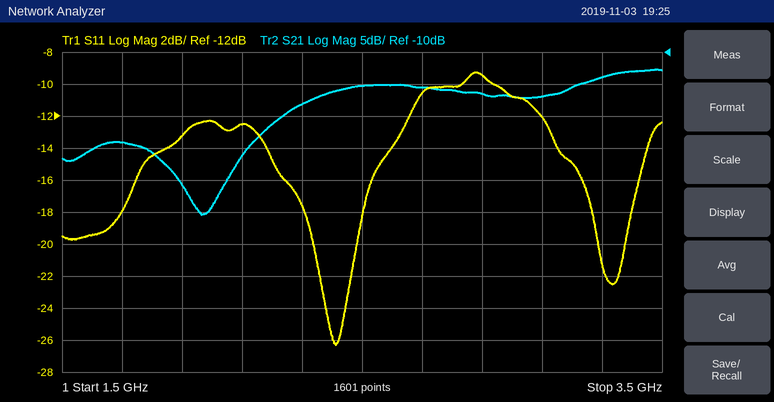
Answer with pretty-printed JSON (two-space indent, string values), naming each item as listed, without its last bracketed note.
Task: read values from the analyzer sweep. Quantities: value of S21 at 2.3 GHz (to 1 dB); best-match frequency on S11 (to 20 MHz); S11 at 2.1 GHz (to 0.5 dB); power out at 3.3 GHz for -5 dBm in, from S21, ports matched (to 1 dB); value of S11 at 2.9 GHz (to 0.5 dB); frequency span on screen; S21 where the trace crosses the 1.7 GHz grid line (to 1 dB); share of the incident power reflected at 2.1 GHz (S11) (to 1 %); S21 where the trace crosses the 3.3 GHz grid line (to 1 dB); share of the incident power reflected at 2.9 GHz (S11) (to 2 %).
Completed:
{
  "value of S21 at 2.3 GHz": "-18 dB",
  "best-match frequency on S11": "2.42 GHz",
  "S11 at 2.1 GHz": "-12.5 dB",
  "power out at 3.3 GHz for -5 dBm in, from S21, ports matched": "-19 dBm",
  "value of S11 at 2.9 GHz": "-9.5 dB",
  "frequency span on screen": "2 GHz",
  "S21 where the trace crosses the 1.7 GHz grid line": "-24 dB",
  "share of the incident power reflected at 2.1 GHz (S11)": "6 %",
  "S21 where the trace crosses the 3.3 GHz grid line": "-14 dB",
  "share of the incident power reflected at 2.9 GHz (S11)": "12 %"
}
